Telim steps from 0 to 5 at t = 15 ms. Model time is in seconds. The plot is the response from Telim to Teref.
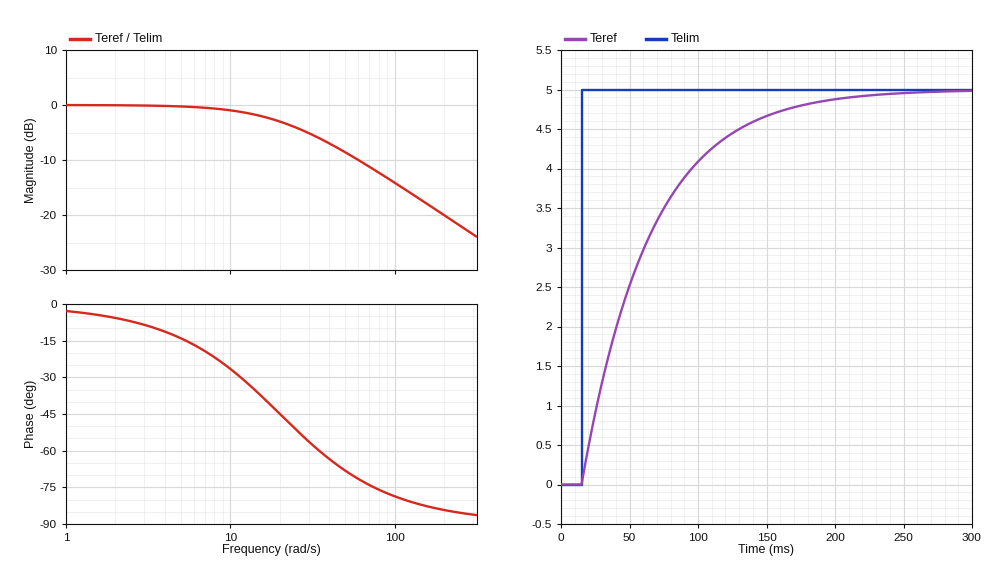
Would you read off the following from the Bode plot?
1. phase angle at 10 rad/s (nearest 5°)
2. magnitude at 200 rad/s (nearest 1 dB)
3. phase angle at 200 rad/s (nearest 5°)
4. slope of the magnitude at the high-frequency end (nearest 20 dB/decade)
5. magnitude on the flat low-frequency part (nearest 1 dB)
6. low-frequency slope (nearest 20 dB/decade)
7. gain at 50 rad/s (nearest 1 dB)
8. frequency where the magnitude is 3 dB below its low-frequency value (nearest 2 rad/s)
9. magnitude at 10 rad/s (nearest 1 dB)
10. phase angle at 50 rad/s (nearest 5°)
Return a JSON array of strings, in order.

["-25°", "-20 dB", "-85°", "-20 dB/decade", "0 dB", "0 dB/decade", "-9 dB", "20 rad/s", "-1 dB", "-70°"]
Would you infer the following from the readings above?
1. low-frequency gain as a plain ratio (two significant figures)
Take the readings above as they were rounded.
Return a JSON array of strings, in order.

["1.0"]
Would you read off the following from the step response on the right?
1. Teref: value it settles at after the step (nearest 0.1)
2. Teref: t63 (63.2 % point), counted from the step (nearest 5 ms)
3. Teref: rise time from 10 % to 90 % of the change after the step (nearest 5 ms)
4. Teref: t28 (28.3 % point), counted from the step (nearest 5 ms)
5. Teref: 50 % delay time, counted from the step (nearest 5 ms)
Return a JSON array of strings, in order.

["5.0", "50 ms", "110 ms", "15 ms", "35 ms"]
